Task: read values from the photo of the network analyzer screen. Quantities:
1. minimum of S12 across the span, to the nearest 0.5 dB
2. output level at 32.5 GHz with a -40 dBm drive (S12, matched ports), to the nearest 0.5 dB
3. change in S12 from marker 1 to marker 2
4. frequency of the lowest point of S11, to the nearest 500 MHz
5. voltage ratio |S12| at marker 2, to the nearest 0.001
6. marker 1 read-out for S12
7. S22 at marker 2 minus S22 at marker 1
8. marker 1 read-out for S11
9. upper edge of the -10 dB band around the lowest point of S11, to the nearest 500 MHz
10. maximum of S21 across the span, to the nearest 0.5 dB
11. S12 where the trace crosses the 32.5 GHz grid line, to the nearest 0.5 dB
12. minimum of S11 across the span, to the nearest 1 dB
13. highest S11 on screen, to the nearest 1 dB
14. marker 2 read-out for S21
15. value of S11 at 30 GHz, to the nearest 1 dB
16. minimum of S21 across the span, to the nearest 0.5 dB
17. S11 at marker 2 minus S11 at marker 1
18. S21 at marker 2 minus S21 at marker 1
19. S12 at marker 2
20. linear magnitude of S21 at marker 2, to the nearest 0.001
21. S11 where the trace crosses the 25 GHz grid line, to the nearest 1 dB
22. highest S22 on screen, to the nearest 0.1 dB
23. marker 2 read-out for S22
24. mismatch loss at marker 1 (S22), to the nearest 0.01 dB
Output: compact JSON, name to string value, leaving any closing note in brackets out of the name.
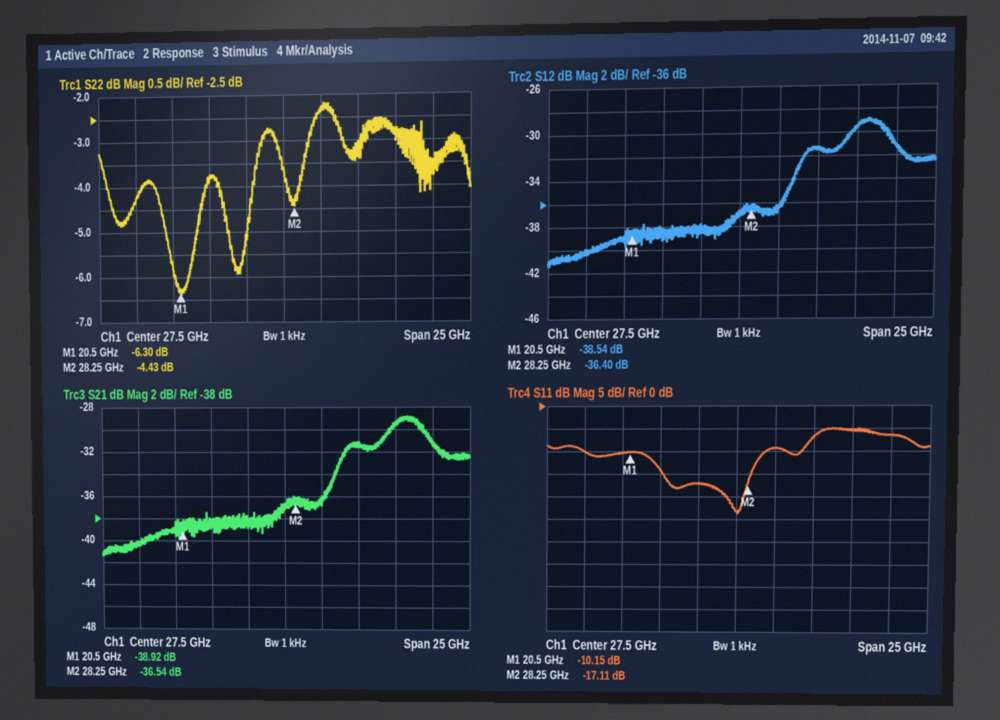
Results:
{"minimum of S12 across the span, to the nearest 0.5 dB": "-41.5 dB", "output level at 32.5 GHz with a -40 dBm drive (S12, matched ports), to the nearest 0.5 dB": "-71.5 dBm", "change in S12 from marker 1 to marker 2": "2.14 dB", "frequency of the lowest point of S11, to the nearest 500 MHz": "27.5 GHz", "voltage ratio |S12| at marker 2, to the nearest 0.001": "0.015", "marker 1 read-out for S12": "-38.54 dB", "S22 at marker 2 minus S22 at marker 1": "1.87 dB", "marker 1 read-out for S11": "-10.15 dB", "upper edge of the -10 dB band around the lowest point of S11, to the nearest 500 MHz": "29.5 GHz", "maximum of S21 across the span, to the nearest 0.5 dB": "-29.0 dB", "S12 where the trace crosses the 32.5 GHz grid line, to the nearest 0.5 dB": "-31.5 dB", "minimum of S11 across the span, to the nearest 1 dB": "-24 dB", "highest S11 on screen, to the nearest 1 dB": "-5 dB", "marker 2 read-out for S21": "-36.54 dB", "value of S11 at 30 GHz, to the nearest 1 dB": "-9 dB", "minimum of S21 across the span, to the nearest 0.5 dB": "-41.5 dB", "S11 at marker 2 minus S11 at marker 1": "-6.96 dB", "S21 at marker 2 minus S21 at marker 1": "2.38 dB", "S12 at marker 2": "-36.40 dB", "linear magnitude of S21 at marker 2, to the nearest 0.001": "0.015", "S11 where the trace crosses the 25 GHz grid line, to the nearest 1 dB": "-17 dB", "highest S22 on screen, to the nearest 0.1 dB": "-2.2 dB", "marker 2 read-out for S22": "-4.43 dB", "mismatch loss at marker 1 (S22), to the nearest 0.01 dB": "1.16 dB"}
